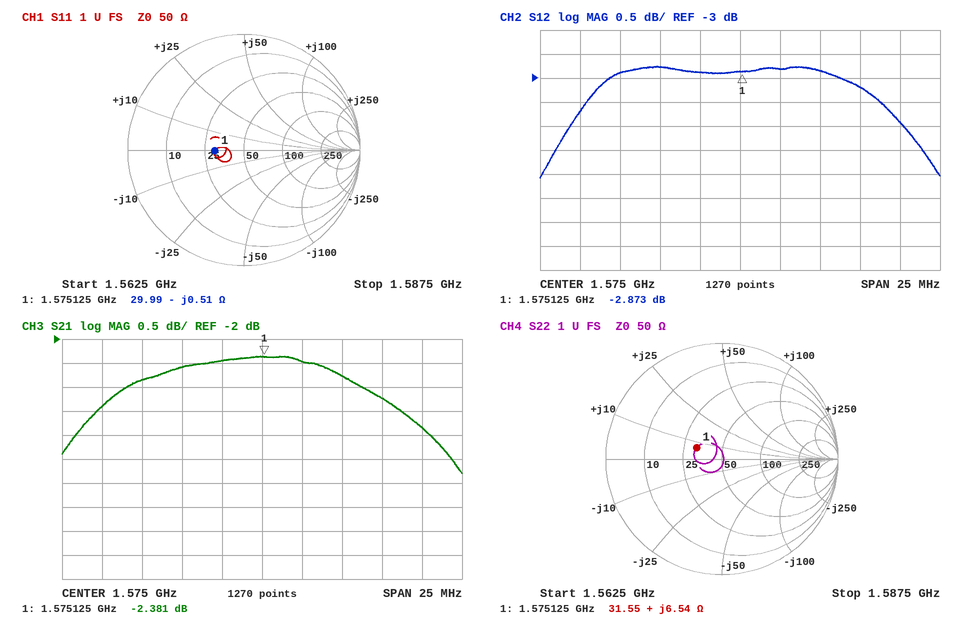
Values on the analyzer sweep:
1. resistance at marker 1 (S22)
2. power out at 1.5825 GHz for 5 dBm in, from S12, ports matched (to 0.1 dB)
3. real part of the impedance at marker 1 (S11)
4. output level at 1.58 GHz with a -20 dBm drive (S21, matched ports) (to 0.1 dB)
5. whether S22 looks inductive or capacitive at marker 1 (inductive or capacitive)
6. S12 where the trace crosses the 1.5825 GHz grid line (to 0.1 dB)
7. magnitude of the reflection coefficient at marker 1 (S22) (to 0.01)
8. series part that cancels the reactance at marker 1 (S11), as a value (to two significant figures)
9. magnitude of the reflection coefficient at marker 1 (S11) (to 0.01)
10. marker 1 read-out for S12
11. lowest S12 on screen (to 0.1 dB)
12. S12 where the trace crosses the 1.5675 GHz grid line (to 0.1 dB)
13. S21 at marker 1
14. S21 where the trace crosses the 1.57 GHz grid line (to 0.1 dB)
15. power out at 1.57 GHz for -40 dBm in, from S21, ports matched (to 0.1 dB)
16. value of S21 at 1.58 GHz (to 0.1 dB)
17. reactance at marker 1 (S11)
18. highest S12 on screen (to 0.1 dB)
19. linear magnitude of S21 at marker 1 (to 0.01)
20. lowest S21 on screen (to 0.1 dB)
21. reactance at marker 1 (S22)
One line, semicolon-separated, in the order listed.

31.55 Ω; 1.8 dBm; 29.99 Ω; -22.8 dBm; inductive; -3.2 dB; 0.24; 52 pH; 0.25; -2.873 dB; -5.1 dB; -2.9 dB; -2.381 dB; -2.6 dB; -42.6 dBm; -2.8 dB; -0.51 Ω; -2.8 dB; 0.76; -4.8 dB; +6.54 Ω
